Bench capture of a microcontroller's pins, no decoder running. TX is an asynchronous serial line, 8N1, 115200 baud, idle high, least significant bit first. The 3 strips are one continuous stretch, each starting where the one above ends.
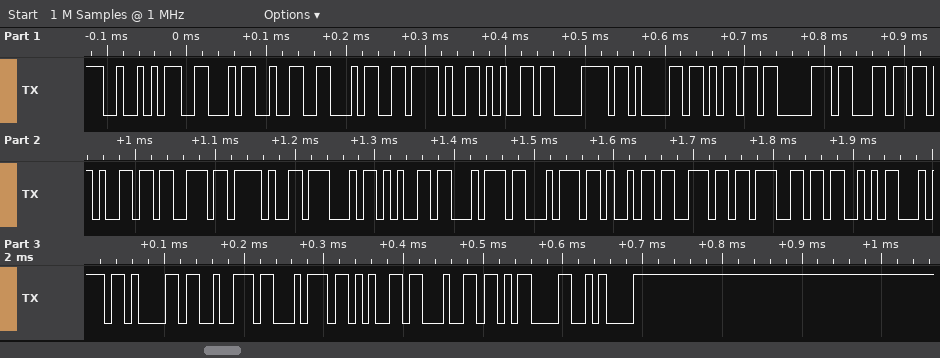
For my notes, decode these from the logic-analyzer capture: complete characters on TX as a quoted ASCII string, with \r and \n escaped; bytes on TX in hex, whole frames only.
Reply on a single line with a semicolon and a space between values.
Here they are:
"RF24/examples/GettingStarted\r\n"; 52 46 32 34 2F 65 78 61 6D 70 6C 65 73 2F 47 65 74 74 69 6E 67 53 74 61 72 74 65 64 0D 0A
